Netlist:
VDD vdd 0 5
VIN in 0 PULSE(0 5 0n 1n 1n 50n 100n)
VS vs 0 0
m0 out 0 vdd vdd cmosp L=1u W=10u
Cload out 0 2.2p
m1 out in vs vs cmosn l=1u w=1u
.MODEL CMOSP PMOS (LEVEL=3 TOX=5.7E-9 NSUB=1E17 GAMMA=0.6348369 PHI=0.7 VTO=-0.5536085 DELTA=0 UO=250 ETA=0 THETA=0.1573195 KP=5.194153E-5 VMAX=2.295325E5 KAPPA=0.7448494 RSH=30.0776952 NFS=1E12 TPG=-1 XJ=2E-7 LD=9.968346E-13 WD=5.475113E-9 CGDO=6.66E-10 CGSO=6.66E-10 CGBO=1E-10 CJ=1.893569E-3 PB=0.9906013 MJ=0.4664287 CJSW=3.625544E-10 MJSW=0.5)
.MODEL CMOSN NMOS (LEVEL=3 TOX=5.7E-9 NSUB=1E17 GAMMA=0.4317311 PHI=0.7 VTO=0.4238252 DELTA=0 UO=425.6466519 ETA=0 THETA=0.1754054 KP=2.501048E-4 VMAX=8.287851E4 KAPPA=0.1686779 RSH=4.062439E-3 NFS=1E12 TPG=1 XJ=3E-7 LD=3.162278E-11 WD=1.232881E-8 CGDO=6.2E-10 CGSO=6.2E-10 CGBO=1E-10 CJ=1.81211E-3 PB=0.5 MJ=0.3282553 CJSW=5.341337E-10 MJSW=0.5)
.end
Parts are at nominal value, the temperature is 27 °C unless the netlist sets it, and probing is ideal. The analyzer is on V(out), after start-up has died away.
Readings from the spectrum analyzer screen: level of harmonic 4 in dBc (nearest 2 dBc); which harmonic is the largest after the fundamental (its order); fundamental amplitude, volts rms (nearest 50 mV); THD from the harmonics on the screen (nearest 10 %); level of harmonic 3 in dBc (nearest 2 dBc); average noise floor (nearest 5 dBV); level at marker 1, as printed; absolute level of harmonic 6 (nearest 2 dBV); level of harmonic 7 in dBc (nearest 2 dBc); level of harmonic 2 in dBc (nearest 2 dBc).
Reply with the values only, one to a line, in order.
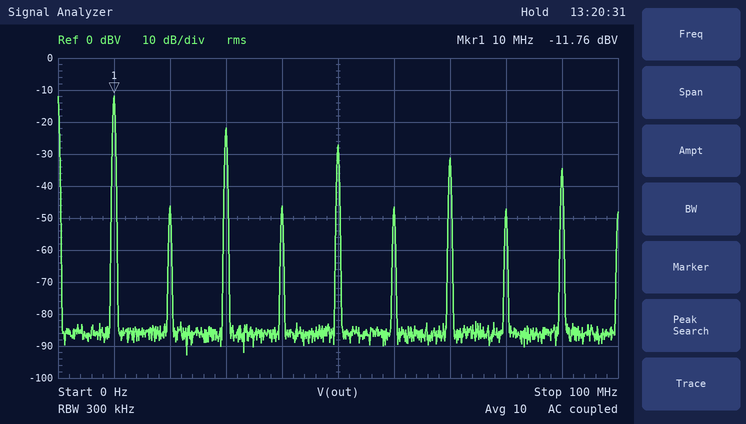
-34 dBc
3
250 mV
40 %
-10 dBc
-85 dBV
-11.76 dBV
-46 dBV
-20 dBc
-34 dBc
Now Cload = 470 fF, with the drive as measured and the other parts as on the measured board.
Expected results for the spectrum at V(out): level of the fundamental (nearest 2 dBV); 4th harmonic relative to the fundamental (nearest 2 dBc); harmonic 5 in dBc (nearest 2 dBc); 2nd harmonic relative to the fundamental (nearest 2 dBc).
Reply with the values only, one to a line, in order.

-12 dBV
-32 dBc
-14 dBc
-32 dBc
